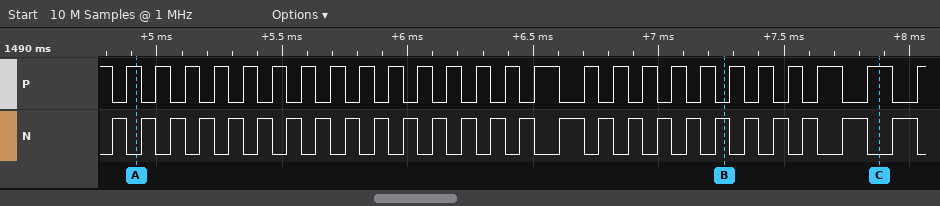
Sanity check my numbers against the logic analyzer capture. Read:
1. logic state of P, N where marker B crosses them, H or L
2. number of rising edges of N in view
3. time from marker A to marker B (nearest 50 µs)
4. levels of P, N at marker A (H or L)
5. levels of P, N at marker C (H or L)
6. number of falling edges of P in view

P=L, N=H
26
2350 µs
P=H, N=L
P=H, N=L
26
